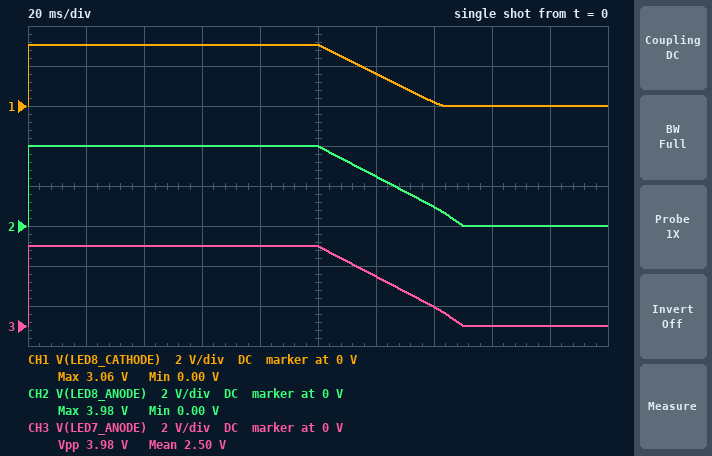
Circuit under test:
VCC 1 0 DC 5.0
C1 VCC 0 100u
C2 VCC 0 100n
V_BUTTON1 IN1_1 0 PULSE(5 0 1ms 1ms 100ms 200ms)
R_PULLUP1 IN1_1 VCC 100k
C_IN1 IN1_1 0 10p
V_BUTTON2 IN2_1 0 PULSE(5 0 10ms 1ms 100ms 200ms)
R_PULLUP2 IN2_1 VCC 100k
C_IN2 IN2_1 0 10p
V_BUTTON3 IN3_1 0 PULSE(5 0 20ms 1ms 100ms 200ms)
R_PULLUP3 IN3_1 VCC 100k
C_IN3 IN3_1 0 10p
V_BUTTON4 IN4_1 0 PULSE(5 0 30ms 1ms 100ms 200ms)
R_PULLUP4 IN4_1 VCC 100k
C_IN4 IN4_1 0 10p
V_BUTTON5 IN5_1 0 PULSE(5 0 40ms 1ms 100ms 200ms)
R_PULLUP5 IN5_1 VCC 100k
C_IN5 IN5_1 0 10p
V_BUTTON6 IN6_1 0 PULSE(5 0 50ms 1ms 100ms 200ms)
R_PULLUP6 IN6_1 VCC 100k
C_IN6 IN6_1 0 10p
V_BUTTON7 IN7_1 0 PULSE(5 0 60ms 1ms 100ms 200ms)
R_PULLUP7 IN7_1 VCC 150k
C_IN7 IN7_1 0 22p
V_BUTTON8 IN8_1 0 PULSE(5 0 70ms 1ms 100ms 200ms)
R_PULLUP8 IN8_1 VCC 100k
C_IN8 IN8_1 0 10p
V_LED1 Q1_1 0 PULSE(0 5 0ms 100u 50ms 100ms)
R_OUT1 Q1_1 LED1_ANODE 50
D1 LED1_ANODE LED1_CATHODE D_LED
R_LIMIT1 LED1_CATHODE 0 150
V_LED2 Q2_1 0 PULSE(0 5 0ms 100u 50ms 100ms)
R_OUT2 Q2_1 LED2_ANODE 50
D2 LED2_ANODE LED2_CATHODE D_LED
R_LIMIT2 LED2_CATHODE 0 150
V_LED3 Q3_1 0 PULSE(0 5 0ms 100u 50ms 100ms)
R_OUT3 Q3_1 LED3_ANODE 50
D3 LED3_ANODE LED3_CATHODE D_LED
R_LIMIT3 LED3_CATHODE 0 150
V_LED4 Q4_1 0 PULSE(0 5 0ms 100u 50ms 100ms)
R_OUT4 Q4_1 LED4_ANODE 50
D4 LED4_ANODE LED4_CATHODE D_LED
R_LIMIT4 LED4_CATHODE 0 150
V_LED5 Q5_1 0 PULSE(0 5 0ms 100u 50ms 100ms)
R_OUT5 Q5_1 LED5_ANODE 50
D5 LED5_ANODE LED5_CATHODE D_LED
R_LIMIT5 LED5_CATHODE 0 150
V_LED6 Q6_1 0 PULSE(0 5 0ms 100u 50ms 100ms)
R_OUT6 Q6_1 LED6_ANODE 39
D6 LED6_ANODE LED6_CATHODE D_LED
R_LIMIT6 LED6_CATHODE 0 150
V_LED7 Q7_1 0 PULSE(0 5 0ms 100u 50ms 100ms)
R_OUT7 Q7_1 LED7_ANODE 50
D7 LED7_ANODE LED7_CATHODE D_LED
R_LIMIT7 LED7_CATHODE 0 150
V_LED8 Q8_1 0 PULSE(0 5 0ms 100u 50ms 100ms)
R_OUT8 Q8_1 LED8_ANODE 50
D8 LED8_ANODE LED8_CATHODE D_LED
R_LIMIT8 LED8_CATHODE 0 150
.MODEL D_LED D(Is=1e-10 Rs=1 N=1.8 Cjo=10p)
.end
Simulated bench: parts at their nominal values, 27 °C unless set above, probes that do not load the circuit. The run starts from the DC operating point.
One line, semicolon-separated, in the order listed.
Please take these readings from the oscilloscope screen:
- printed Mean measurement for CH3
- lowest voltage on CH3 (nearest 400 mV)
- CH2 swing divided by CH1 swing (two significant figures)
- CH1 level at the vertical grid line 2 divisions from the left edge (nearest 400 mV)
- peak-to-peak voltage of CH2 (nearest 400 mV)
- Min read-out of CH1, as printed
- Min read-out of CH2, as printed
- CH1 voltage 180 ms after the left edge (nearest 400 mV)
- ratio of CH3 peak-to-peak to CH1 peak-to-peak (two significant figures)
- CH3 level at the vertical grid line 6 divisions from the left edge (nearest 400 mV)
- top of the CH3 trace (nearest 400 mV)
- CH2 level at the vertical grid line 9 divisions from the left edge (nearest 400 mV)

2.50 V; 0 V; 1.3; 3.2 V; 4.0 V; 0.00 V; 0.00 V; 0 V; 1.3; 2.4 V; 4.0 V; 0 V
